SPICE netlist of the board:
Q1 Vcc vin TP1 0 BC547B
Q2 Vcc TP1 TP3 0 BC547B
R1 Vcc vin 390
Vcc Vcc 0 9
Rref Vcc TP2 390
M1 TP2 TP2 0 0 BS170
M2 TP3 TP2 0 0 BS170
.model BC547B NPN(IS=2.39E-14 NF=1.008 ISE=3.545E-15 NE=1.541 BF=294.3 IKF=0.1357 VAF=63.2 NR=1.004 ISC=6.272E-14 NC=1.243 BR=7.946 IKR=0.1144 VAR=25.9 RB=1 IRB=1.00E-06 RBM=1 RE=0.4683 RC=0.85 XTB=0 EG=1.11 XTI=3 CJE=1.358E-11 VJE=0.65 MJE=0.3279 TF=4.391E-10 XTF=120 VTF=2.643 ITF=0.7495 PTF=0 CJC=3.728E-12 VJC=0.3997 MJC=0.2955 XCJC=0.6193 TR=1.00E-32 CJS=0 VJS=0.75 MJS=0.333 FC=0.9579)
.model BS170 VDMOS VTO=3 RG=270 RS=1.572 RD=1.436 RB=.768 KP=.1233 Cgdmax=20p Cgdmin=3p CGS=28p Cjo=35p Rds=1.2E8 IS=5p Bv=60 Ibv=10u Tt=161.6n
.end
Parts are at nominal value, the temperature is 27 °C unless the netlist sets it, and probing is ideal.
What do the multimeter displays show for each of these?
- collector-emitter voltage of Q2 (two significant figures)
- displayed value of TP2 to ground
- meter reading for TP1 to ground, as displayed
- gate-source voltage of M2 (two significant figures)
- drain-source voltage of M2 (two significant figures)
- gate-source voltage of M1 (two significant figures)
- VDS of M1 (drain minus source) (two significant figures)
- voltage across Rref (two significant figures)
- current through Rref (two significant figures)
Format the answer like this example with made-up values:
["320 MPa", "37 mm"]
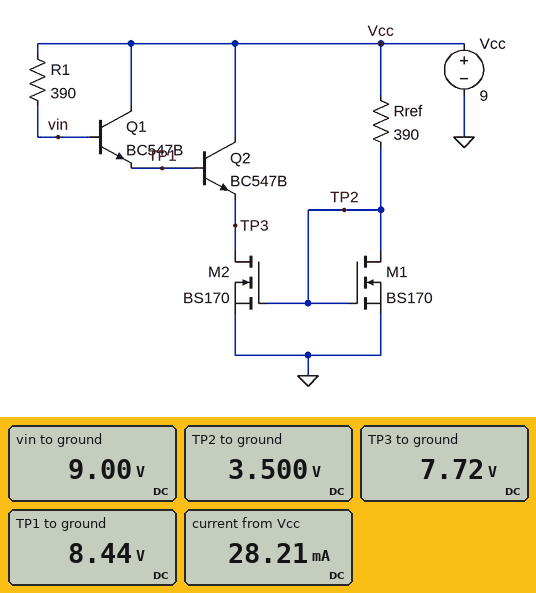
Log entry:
["1.3 V", "3.500 V", "8.44 V", "3.5 V", "7.7 V", "3.5 V", "3.5 V", "5.5 V", "14 mA"]
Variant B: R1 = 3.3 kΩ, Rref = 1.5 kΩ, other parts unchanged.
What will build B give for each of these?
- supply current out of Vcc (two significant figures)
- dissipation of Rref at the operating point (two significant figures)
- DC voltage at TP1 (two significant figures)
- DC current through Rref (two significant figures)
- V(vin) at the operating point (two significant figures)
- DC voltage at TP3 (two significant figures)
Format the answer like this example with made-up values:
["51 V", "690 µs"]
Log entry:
["7.7 mA", "22 mW", "8.5 V", "3.8 mA", "9.0 V", "7.8 V"]
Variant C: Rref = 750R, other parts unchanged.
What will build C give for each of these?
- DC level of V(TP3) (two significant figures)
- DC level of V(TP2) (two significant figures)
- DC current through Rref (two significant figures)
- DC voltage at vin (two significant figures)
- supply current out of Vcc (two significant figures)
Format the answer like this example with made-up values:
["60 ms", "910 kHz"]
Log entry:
["7.8 V", "3.4 V", "7.5 mA", "9.0 V", "15 mA"]
